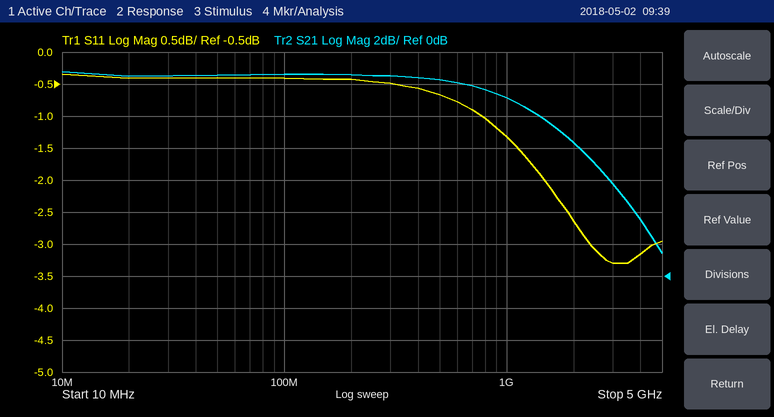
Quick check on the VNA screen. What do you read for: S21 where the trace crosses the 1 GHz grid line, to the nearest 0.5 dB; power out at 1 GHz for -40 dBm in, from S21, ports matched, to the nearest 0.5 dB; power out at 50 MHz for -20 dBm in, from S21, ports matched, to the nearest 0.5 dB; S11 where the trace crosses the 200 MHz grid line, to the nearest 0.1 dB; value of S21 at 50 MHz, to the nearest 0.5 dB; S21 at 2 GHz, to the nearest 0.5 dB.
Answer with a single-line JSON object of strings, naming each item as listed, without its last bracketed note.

{"S21 where the trace crosses the 1 GHz grid line, to the nearest 0.5 dB": "11.0 dB", "power out at 1 GHz for -40 dBm in, from S21, ports matched, to the nearest 0.5 dB": "-29.0 dBm", "power out at 50 MHz for -20 dBm in, from S21, ports matched, to the nearest 0.5 dB": "-7.5 dBm", "S11 where the trace crosses the 200 MHz grid line, to the nearest 0.1 dB": "-0.4 dB", "value of S21 at 50 MHz, to the nearest 0.5 dB": "12.5 dB", "S21 at 2 GHz, to the nearest 0.5 dB": "8.5 dB"}
